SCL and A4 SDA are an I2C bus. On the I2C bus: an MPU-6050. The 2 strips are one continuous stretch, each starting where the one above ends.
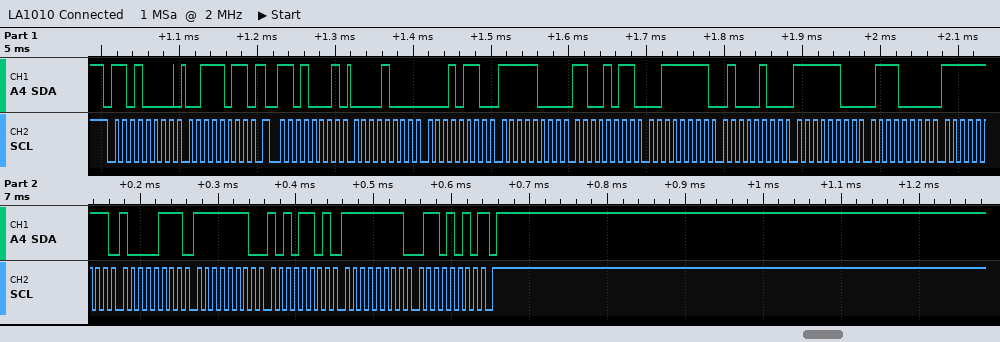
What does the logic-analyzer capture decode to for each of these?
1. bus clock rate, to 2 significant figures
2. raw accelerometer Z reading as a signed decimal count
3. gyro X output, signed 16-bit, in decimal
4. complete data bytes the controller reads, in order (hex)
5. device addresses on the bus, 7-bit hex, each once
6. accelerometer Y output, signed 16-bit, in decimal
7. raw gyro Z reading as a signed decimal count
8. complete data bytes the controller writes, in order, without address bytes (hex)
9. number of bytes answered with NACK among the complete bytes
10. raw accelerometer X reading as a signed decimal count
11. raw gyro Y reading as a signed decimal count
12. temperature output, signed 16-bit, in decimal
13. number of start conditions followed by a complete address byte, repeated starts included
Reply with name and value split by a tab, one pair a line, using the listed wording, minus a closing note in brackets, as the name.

bus clock rate, to 2 significant figures	100 kHz
raw accelerometer Z reading as a signed decimal count	16196
gyro X output, signed 16-bit, in decimal	-121
complete data bytes the controller reads, in order	08 16 F8 CB 3F 44 FC 70 FF 87 FE AD FF 6A
device addresses on the bus, 7-bit hex, each once	0x68
accelerometer Y output, signed 16-bit, in decimal	-1845
raw gyro Z reading as a signed decimal count	-150
complete data bytes the controller writes, in order, without address bytes	3B
number of bytes answered with NACK among the complete bytes	1
raw accelerometer X reading as a signed decimal count	2070
raw gyro Y reading as a signed decimal count	-339
temperature output, signed 16-bit, in decimal	-912
number of start conditions followed by a complete address byte, repeated starts included	2
